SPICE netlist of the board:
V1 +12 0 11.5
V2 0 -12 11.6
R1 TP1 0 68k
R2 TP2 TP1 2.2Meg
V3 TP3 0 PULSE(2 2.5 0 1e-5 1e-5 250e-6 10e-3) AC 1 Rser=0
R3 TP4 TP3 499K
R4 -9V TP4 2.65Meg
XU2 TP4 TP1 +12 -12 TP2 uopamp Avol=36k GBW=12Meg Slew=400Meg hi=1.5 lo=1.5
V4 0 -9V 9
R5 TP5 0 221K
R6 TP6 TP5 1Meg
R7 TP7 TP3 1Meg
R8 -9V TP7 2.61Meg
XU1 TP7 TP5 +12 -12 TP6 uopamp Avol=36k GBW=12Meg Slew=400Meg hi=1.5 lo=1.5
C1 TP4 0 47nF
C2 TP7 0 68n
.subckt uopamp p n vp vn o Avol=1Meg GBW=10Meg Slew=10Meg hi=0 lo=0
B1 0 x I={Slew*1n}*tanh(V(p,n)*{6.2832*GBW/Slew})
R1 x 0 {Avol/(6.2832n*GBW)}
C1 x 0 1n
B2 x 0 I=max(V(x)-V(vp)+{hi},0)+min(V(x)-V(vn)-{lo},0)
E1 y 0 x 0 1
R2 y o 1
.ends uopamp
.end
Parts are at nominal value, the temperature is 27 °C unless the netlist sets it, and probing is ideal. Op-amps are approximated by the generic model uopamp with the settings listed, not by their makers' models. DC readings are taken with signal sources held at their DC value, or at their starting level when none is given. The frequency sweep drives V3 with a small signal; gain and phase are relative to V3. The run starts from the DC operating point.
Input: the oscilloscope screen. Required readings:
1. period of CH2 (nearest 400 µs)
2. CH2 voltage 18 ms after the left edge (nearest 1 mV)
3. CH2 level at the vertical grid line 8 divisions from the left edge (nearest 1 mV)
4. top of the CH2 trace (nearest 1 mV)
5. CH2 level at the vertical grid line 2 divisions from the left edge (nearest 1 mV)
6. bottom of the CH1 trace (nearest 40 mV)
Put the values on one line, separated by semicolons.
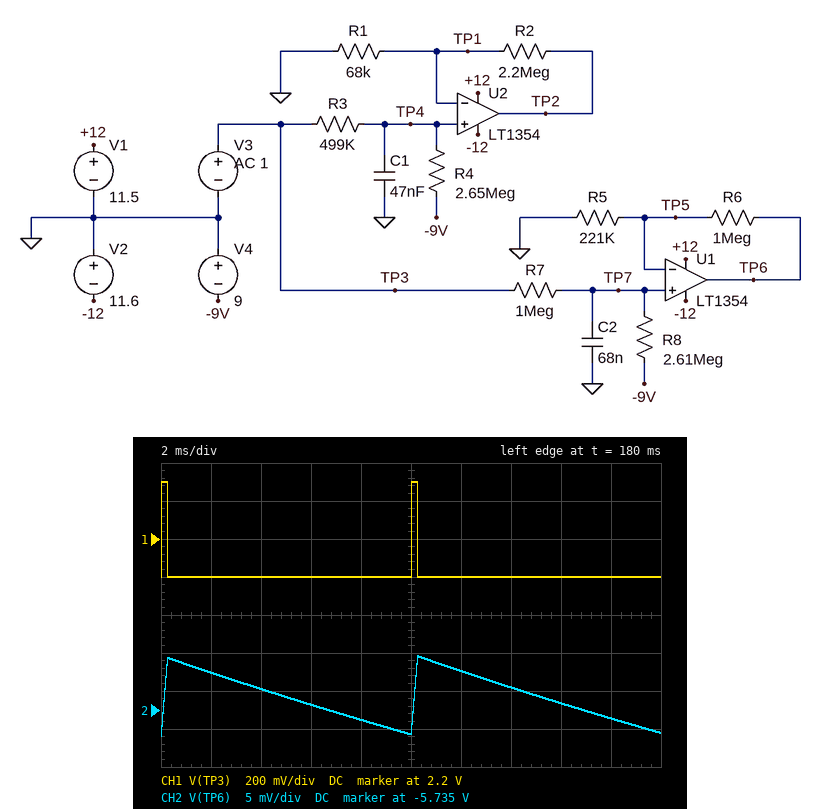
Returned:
10.0 ms; -5.736 V; -5.734 V; -5.728 V; -5.732 V; 2.00 V
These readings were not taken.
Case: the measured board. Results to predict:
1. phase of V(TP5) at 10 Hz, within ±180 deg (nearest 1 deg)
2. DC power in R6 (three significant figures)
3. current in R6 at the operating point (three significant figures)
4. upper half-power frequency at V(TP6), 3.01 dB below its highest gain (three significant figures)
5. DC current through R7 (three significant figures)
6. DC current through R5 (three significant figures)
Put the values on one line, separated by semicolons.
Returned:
-72 deg; 22.4 µW; 4.74 µA; 3.24 Hz; 3.05 µA; 4.74 µA
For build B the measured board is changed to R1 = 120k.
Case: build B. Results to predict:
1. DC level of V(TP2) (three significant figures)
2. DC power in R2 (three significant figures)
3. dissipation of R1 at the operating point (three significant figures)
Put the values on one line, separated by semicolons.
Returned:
4.96 V; 10.1 µW; 549 nW
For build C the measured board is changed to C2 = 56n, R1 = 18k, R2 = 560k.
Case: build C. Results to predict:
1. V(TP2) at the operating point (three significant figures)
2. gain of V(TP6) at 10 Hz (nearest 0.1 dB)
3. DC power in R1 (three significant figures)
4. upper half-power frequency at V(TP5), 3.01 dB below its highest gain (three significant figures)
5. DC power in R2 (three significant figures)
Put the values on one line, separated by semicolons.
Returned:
8.24 V; 3.3 dB; 3.66 µW; 3.93 Hz; 114 µW
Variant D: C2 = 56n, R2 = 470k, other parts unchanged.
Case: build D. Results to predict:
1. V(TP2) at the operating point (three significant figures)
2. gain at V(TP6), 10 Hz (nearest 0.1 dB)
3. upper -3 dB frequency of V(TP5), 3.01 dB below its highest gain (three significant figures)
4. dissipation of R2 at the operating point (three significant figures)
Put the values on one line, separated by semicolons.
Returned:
2.03 V; 3.3 dB; 3.93 Hz; 6.71 µW
